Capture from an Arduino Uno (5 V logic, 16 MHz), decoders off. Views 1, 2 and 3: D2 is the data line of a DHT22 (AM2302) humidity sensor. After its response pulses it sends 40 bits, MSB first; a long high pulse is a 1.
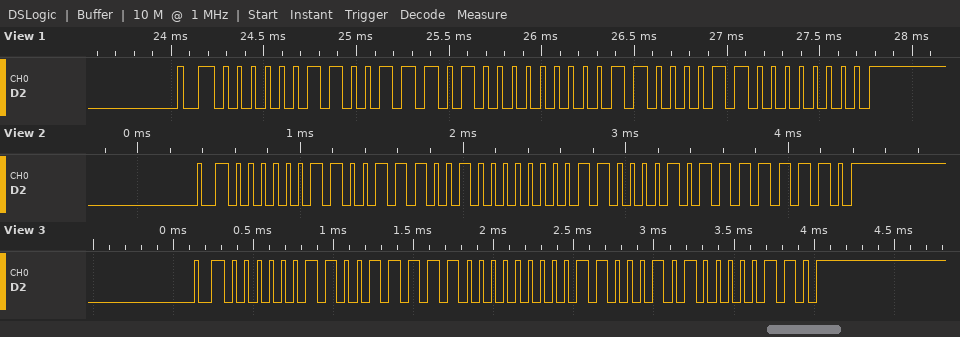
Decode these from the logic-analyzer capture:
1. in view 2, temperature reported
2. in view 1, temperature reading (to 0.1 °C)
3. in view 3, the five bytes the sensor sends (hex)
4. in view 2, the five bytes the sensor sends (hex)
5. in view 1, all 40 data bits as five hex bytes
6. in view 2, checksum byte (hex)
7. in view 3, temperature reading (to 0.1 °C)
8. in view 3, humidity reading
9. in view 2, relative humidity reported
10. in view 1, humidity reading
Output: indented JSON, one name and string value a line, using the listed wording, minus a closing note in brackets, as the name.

{
  "in view 2, temperature reported": "19.4 °C",
  "in view 1, temperature reading": "19.5 °C",
  "in view 3, the five bytes the sensor sends": "03 3E 00 C5 06",
  "in view 2, the five bytes the sensor sends": "03 39 00 C2 FE",
  "in view 1, all 40 data bits as five hex bytes": "03 3A 00 C3 00",
  "in view 2, checksum byte": "0xFE",
  "in view 3, temperature reading": "19.7 °C",
  "in view 3, humidity reading": "83.0 %",
  "in view 2, relative humidity reported": "82.5 %",
  "in view 1, humidity reading": "82.6 %"
}
